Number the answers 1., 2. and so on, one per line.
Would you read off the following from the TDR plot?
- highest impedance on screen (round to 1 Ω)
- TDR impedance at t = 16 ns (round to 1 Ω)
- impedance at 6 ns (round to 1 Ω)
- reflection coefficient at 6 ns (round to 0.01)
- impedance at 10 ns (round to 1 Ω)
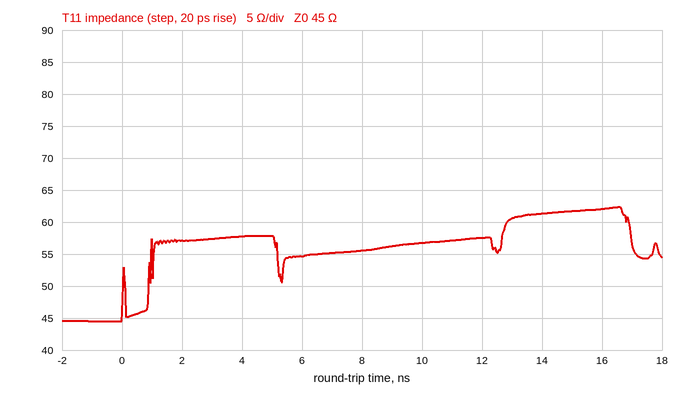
1. 62 Ω
2. 62 Ω
3. 55 Ω
4. +0.10
5. 57 Ω
